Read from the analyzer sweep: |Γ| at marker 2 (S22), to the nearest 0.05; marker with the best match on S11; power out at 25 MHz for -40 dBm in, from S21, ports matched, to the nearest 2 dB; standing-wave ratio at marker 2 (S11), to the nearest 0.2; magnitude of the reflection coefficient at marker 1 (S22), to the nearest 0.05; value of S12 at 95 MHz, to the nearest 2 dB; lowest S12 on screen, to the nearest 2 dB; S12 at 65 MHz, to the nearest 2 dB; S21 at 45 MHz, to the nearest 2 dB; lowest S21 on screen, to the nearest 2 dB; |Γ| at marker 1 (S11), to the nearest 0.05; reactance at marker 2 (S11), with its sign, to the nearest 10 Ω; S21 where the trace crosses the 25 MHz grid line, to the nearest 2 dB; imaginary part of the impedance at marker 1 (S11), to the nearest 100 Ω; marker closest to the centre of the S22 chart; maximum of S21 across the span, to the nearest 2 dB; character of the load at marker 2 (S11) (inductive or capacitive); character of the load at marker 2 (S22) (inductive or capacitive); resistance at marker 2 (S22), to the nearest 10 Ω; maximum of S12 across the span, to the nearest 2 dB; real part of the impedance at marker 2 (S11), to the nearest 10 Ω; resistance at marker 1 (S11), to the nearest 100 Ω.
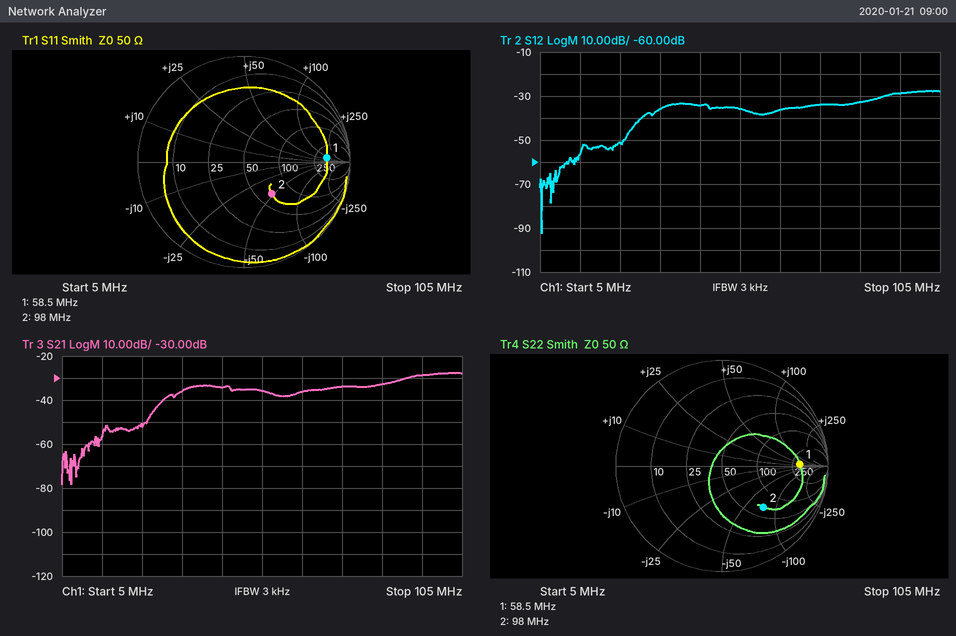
0.55
marker 2
-92 dBm
2.4
0.75
-28 dB
-92 dB
-36 dB
-34 dB
-78 dB
0.80
-50 Ω
-52 dB
+100 Ω
marker 2
-28 dB
capacitive
capacitive
70 Ω
-28 dB
70 Ω
400 Ω
